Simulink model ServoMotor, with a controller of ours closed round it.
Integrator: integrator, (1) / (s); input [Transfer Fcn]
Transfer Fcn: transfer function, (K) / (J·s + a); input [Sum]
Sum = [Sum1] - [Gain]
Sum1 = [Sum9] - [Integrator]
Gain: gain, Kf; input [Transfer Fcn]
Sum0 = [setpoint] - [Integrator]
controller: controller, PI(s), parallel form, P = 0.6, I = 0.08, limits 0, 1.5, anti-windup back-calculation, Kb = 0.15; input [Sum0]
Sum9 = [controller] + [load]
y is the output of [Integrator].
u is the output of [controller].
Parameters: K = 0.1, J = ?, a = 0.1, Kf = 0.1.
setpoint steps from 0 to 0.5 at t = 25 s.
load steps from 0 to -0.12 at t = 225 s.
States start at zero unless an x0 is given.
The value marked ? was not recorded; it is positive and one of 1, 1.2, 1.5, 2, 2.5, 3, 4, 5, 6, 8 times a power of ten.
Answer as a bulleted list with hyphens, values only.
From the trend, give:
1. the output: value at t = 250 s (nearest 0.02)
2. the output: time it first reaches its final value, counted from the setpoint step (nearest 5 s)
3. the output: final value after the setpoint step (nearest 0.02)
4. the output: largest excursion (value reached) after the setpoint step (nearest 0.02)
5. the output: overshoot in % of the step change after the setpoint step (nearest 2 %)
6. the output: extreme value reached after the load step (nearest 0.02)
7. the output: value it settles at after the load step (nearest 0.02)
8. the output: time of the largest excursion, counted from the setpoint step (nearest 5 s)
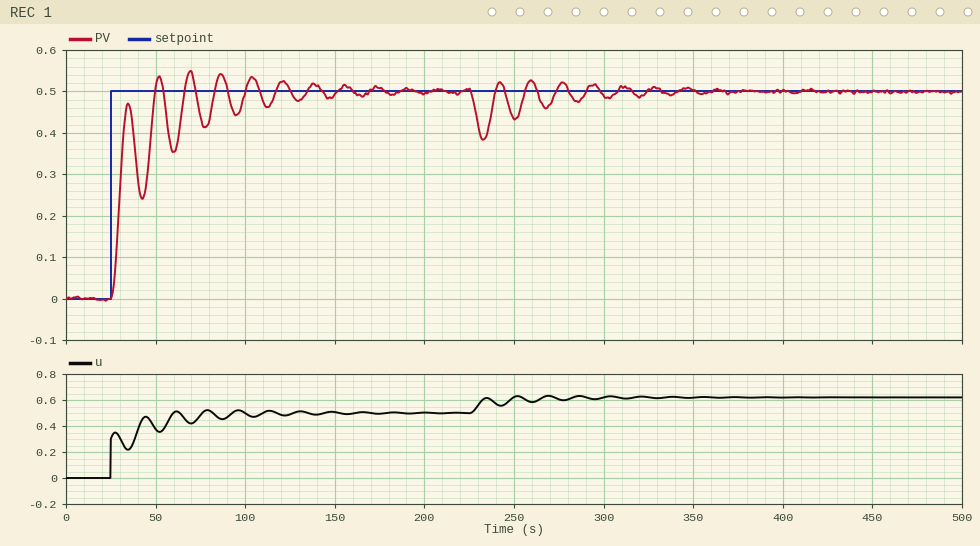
- 0.44
- 25 s
- 0.50
- 0.54
- 10 %
- 0.38
- 0.50
- 45 s
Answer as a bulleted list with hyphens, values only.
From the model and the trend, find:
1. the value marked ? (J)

- 1.2
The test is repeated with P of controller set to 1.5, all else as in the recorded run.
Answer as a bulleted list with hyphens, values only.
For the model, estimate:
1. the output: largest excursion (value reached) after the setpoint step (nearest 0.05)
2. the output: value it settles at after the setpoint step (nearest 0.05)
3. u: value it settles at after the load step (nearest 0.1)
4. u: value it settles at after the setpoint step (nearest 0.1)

- 0.60
- 0.50
- 0.6
- 0.5
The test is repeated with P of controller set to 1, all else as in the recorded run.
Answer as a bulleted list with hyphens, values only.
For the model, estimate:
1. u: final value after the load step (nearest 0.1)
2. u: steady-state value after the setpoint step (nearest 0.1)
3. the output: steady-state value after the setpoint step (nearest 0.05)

- 0.6
- 0.5
- 0.50
